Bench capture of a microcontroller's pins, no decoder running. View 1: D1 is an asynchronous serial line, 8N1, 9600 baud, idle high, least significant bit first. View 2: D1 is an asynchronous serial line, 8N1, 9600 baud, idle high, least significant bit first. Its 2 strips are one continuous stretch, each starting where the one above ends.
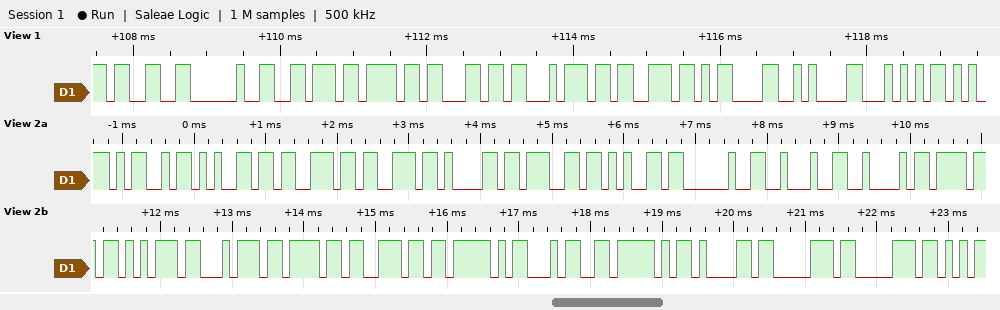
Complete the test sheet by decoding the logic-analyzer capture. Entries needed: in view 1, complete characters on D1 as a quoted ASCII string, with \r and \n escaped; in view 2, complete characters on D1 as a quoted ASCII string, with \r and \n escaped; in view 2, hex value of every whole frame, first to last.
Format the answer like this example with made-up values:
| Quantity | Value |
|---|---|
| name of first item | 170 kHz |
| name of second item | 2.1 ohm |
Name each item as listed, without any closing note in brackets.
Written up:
| Quantity | Value |
|---|---|
| in view 1, complete characters on D1 as a quoted ASCII string, with \r and \n escaped | "3 volts\r\nT" |
| in view 2, complete characters on D1 as a quoted ASCII string, with \r and \n escaped | "Message \"Bouton_4_app" |
| in view 2, hex value of every whole frame, first to last | 4D 65 73 73 61 67 65 20 22 42 6F 75 74 6F 6E 5F 34 5F 61 70 70 |
